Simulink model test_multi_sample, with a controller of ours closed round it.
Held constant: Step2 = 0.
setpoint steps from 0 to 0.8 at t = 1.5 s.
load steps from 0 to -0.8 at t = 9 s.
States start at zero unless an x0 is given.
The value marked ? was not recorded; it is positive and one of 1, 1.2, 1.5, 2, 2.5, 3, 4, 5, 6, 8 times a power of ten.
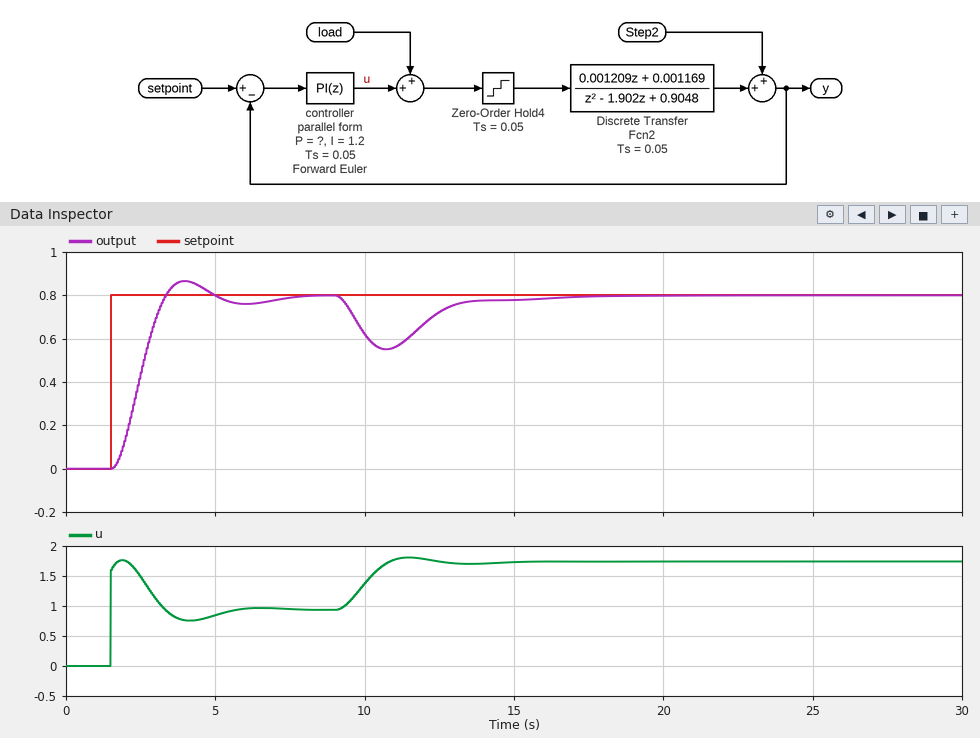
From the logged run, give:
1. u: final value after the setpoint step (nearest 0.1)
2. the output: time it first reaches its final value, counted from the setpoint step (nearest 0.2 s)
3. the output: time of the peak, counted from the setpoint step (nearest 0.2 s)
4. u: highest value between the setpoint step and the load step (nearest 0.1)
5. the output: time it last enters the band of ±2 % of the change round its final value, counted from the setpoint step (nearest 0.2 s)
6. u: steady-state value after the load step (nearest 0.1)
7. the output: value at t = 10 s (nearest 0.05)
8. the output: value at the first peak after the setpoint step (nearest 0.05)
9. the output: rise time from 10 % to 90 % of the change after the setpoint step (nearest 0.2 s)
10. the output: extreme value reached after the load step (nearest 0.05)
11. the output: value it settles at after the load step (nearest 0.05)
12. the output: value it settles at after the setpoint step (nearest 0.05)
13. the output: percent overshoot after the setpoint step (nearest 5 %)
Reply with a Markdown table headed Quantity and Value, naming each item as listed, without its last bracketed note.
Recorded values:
| Quantity | Value |
|---|---|
| u: final value after the setpoint step | 0.9 |
| the output: time it first reaches its final value, counted from the setpoint step | 1.8 s |
| the output: time of the peak, counted from the setpoint step | 2.4 s |
| u: highest value between the setpoint step and the load step | 1.8 |
| the output: time it last enters the band of ±2 % of the change round its final value, counted from the setpoint step | 5.8 s |
| u: steady-state value after the load step | 1.7 |
| the output: value at t = 10 s | 0.60 |
| the output: value at the first peak after the setpoint step | 0.85 |
| the output: rise time from 10 % to 90 % of the change after the setpoint step | 1.2 s |
| the output: extreme value reached after the load step | 0.55 |
| the output: value it settles at after the load step | 0.80 |
| the output: value it settles at after the setpoint step | 0.80 |
| the output: percent overshoot after the setpoint step | 10 % |
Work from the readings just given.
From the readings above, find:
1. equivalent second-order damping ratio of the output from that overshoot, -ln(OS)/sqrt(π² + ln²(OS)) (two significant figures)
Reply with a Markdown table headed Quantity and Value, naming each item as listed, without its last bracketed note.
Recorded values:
| Quantity | Value |
|---|---|
| equivalent second-order damping ratio of the output from that overshoot, -ln(OS)/sqrt(π² + ln²(OS)) | 0.59 |
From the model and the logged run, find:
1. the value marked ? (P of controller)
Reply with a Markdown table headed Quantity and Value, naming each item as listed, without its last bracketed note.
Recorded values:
| Quantity | Value |
|---|---|
| the value marked ? | 2 |
